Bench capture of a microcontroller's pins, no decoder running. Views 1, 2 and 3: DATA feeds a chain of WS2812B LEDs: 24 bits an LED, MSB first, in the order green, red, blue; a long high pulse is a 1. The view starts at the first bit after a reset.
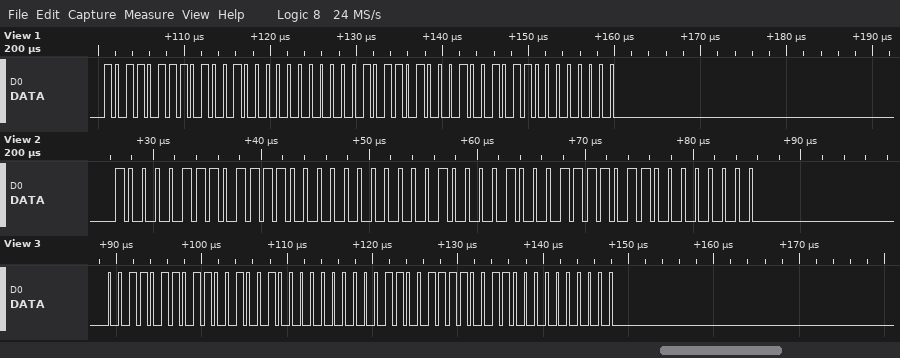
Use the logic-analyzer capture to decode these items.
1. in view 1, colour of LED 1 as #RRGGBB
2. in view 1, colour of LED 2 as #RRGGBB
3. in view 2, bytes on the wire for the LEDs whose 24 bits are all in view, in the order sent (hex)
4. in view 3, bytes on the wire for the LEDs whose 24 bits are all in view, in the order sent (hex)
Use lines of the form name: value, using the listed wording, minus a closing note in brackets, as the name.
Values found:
in view 1, colour of LED 1 as #RRGGBB: #48B700
in view 1, colour of LED 2 as #RRGGBB: #4BB400
in view 2, bytes on the wire for the LEDs whose 24 bits are all in view, in the order sent: 87 78 00 84 7B 00
in view 3, bytes on the wire for the LEDs whose 24 bits are all in view, in the order sent: 36 C9 00 33 CC 00
